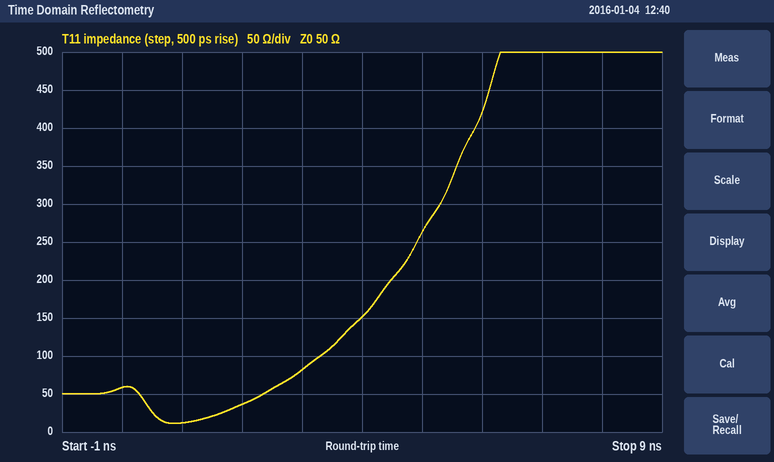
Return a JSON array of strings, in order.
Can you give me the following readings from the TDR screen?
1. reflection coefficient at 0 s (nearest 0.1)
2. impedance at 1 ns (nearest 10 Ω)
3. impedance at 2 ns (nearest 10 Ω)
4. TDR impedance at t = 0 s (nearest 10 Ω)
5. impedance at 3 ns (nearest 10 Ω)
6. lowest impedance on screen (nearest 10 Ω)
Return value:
["+0.1", "10 Ω", "40 Ω", "60 Ω", "80 Ω", "10 Ω"]
